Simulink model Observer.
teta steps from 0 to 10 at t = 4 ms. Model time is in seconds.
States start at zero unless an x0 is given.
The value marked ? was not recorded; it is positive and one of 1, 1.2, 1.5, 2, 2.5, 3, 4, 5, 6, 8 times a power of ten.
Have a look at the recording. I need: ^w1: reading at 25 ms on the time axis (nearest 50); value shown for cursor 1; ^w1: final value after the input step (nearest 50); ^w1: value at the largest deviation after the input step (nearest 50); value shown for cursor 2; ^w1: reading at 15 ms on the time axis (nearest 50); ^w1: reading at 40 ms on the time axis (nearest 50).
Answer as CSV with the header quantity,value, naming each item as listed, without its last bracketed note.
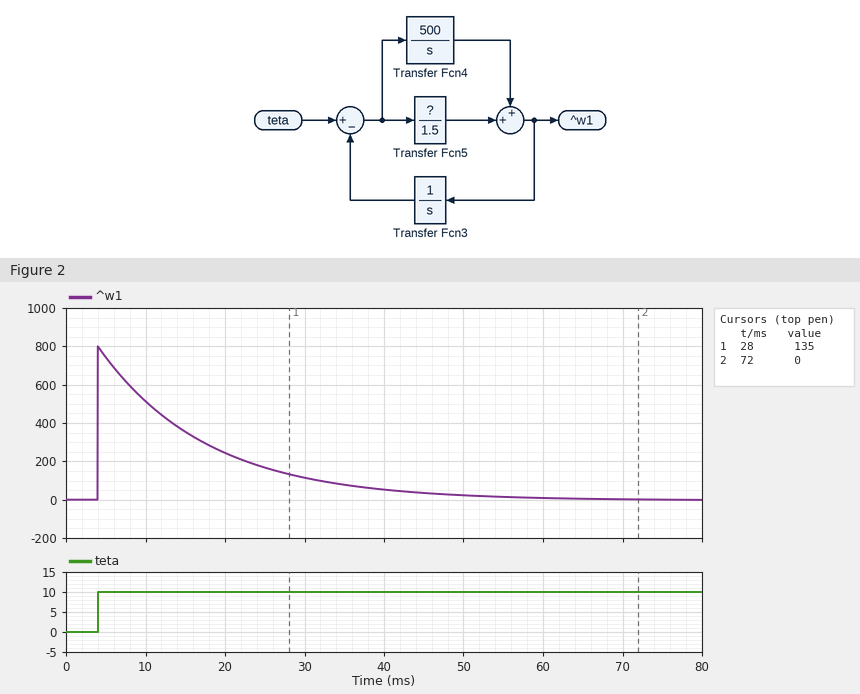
quantity,value
^w1: reading at 25 ms on the time axis,150
value shown for cursor 1,135
^w1: final value after the input step,0
^w1: value at the largest deviation after the input step,800
value shown for cursor 2,0
^w1: reading at 15 ms on the time axis,350
^w1: reading at 40 ms on the time axis,50
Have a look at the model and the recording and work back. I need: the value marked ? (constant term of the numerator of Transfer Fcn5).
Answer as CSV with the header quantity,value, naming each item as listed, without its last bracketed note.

quantity,value
the value marked ?,120
